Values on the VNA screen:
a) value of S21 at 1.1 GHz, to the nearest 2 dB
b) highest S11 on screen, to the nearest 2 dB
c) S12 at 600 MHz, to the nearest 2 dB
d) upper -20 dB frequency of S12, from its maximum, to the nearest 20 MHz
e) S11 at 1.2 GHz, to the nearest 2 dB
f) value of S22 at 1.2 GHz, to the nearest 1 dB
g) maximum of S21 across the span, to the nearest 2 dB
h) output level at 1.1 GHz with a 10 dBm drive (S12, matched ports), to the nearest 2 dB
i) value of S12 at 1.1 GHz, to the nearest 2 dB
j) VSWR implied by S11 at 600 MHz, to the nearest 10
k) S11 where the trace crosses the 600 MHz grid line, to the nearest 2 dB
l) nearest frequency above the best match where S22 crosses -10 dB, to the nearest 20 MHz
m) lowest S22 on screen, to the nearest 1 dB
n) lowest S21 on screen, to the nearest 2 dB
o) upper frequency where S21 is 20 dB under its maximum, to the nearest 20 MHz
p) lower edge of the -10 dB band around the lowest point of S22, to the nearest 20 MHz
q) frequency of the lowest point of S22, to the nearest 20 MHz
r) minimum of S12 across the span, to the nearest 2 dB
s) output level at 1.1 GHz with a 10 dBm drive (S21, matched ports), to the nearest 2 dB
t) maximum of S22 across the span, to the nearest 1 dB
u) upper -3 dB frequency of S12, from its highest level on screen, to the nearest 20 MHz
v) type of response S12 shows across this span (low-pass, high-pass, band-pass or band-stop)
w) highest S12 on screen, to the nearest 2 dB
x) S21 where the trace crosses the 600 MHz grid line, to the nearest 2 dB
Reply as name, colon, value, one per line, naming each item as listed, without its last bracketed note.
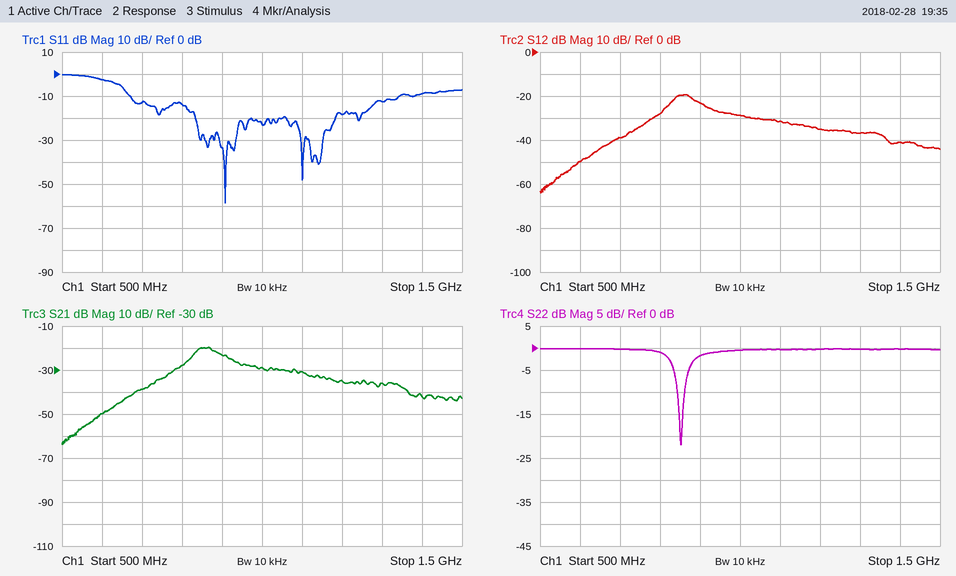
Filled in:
value of S21 at 1.1 GHz, to the nearest 2 dB: -30 dB
highest S11 on screen, to the nearest 2 dB: 0 dB
S12 at 600 MHz, to the nearest 2 dB: -50 dB
upper -20 dB frequency of S12, from its maximum, to the nearest 20 MHz: 1.36 GHz
S11 at 1.2 GHz, to the nearest 2 dB: -18 dB
value of S22 at 1.2 GHz, to the nearest 1 dB: 0 dB
maximum of S21 across the span, to the nearest 2 dB: -20 dB
output level at 1.1 GHz with a 10 dBm drive (S12, matched ports), to the nearest 2 dB: -22 dBm
value of S12 at 1.1 GHz, to the nearest 2 dB: -32 dB
VSWR implied by S11 at 600 MHz, to the nearest 10: 10
S11 where the trace crosses the 600 MHz grid line, to the nearest 2 dB: -2 dB
nearest frequency above the best match where S22 crosses -10 dB, to the nearest 20 MHz: 860 MHz
lowest S22 on screen, to the nearest 1 dB: -22 dB
lowest S21 on screen, to the nearest 2 dB: -64 dB
upper frequency where S21 is 20 dB under its maximum, to the nearest 20 MHz: 1.36 GHz
lower edge of the -10 dB band around the lowest point of S22, to the nearest 20 MHz: 840 MHz
frequency of the lowest point of S22, to the nearest 20 MHz: 860 MHz
minimum of S12 across the span, to the nearest 2 dB: -64 dB
output level at 1.1 GHz with a 10 dBm drive (S21, matched ports), to the nearest 2 dB: -20 dBm
maximum of S22 across the span, to the nearest 1 dB: 0 dB
upper -3 dB frequency of S12, from its highest level on screen, to the nearest 20 MHz: 900 MHz
type of response S12 shows across this span: band-pass
highest S12 on screen, to the nearest 2 dB: -20 dB
S21 where the trace crosses the 600 MHz grid line, to the nearest 2 dB: -50 dB
